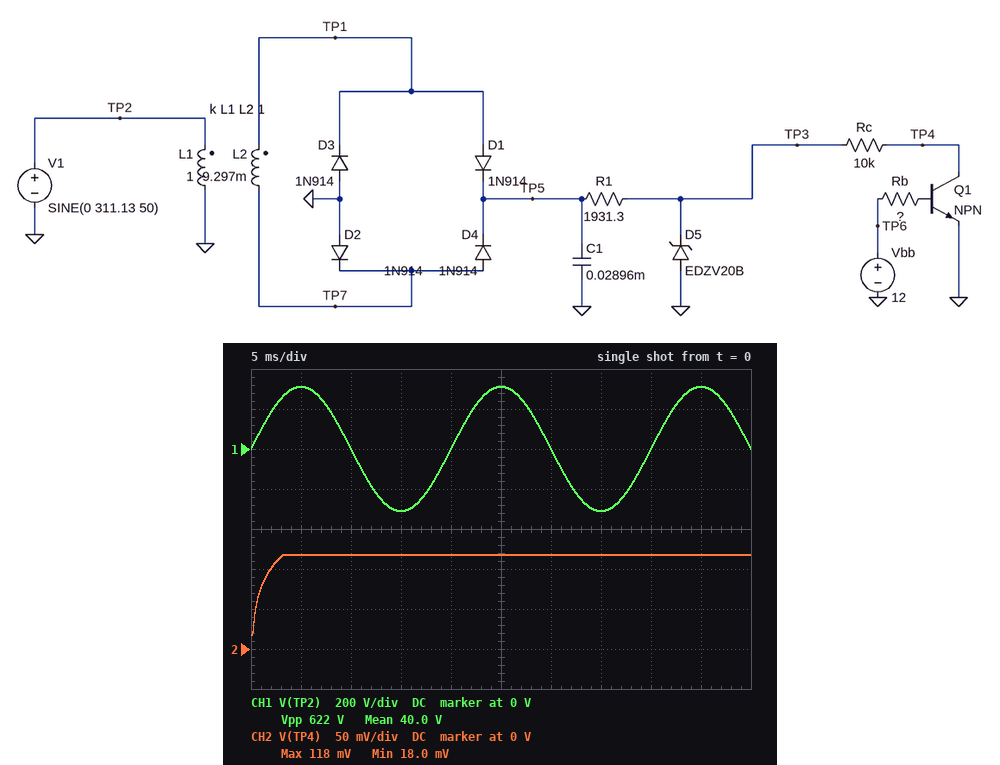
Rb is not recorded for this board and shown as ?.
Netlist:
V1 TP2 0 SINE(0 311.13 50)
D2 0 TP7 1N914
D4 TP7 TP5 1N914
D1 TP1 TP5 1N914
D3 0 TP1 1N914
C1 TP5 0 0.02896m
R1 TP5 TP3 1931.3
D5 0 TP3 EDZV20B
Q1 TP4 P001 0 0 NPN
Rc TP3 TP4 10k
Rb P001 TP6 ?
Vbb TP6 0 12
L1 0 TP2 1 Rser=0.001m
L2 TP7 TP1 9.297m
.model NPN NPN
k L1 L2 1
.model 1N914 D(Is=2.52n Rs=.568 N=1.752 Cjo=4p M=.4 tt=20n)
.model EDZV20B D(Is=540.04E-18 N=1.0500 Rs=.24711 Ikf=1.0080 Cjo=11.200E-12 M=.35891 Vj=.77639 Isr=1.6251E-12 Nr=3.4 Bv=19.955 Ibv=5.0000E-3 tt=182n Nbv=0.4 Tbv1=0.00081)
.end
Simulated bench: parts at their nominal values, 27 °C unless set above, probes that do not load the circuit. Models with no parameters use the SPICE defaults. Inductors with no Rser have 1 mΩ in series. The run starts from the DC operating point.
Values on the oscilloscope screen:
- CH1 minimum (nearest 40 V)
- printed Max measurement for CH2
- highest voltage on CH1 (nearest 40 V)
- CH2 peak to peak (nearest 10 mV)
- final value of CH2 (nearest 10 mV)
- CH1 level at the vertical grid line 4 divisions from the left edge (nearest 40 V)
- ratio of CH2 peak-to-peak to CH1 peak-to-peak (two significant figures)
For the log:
-320 V
118 mV
320 V
100 mV
120 mV
0 V
0.00016
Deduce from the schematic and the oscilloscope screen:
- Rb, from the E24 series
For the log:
270 kΩ
